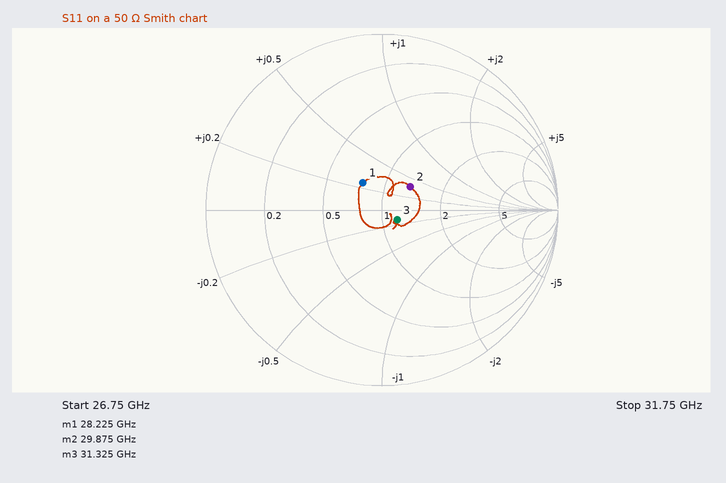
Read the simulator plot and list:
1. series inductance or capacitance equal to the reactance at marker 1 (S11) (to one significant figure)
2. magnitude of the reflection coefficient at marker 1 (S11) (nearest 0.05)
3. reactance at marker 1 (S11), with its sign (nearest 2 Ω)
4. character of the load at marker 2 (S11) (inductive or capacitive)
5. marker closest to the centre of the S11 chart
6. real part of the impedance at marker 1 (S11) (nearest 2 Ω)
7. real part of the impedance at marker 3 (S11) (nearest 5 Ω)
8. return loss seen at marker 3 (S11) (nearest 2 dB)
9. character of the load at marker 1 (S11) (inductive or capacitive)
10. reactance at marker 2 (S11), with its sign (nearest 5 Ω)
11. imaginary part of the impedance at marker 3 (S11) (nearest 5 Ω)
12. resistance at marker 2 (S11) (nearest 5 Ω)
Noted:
70 pH
0.20
+12 Ω
inductive
marker 3
38 Ω
60 Ω
20 dB
inductive
+20 Ω
-5 Ω
65 Ω
